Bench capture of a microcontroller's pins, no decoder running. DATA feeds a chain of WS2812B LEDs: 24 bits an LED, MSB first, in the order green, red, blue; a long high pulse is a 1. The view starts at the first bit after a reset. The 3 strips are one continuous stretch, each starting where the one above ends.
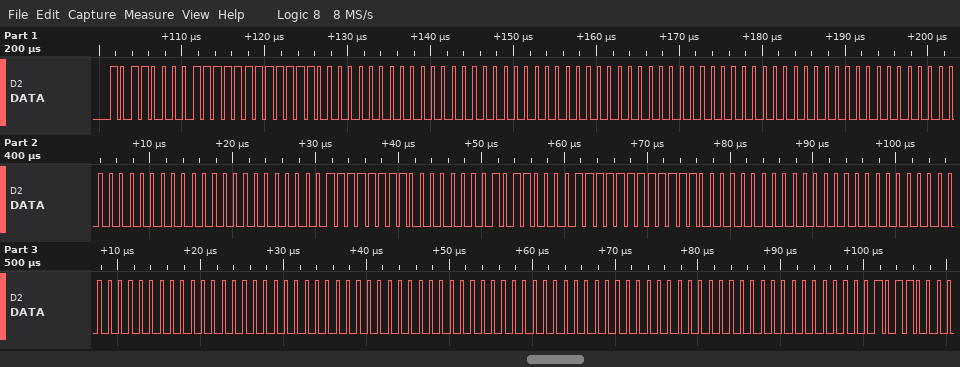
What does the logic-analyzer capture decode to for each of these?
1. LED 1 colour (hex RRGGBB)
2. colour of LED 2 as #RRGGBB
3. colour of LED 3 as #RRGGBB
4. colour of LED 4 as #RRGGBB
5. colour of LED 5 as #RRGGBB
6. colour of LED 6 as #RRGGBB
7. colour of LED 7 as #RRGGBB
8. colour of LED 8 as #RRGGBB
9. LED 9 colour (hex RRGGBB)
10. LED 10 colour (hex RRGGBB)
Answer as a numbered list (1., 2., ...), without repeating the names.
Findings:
1. #FFB0F0
2. #000000
3. #000000
4. #000000
5. #FF0000
6. #FFB0F0
7. #000000
8. #000000
9. #000000
10. #000000
